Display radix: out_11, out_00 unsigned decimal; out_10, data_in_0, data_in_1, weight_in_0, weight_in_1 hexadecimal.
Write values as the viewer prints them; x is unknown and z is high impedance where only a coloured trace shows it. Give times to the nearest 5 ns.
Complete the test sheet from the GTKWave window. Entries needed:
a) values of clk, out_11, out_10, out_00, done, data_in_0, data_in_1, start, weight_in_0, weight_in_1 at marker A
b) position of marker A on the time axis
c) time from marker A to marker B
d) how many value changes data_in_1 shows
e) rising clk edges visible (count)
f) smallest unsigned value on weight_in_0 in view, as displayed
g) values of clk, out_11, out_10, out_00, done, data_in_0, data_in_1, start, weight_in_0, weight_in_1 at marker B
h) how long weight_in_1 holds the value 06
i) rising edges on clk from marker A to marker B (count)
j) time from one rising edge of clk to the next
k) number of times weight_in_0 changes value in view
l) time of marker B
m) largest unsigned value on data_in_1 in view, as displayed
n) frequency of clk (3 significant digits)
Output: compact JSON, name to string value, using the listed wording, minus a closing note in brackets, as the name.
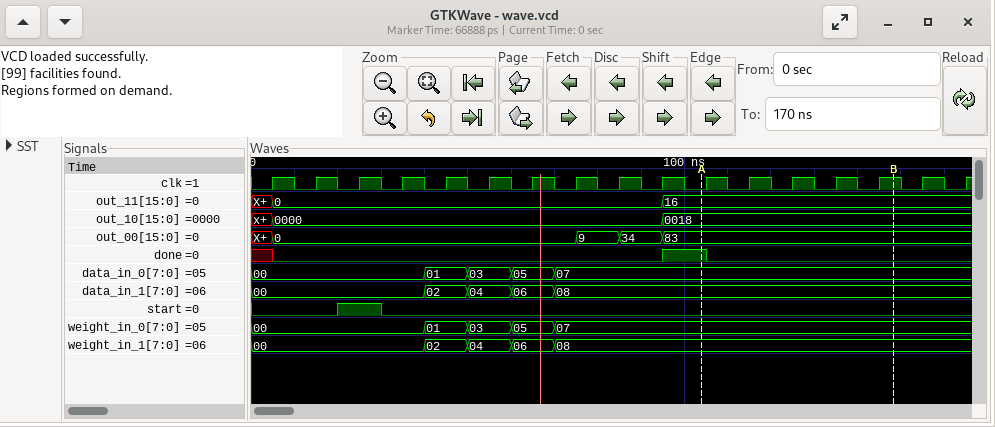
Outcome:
{"values of clk, out_11, out_10, out_00, done, data_in_0, data_in_1, start, weight_in_0, weight_in_1 at marker A": "clk=0, out_11=16, out_10=0018, out_00=83, done=1, data_in_0=07, data_in_1=08, start=0, weight_in_0=07, weight_in_1=08", "position of marker A on the time axis": "105 ns", "time from marker A to marker B": "45 ns", "how many value changes data_in_1 shows": "4", "rising clk edges visible": "17", "smallest unsigned value on weight_in_0 in view, as displayed": "00", "values of clk, out_11, out_10, out_00, done, data_in_0, data_in_1, start, weight_in_0, weight_in_1 at marker B": "clk=1, out_11=16, out_10=0018, out_00=83, done=0, data_in_0=07, data_in_1=08, start=0, weight_in_0=07, weight_in_1=08", "how long weight_in_1 holds the value 06": "10 ns", "rising edges on clk from marker A to marker B": "5", "time from one rising edge of clk to the next": "10 ns", "number of times weight_in_0 changes value in view": "4", "time of marker B": "150 ns", "largest unsigned value on data_in_1 in view, as displayed": "08", "frequency of clk": "100 MHz"}
